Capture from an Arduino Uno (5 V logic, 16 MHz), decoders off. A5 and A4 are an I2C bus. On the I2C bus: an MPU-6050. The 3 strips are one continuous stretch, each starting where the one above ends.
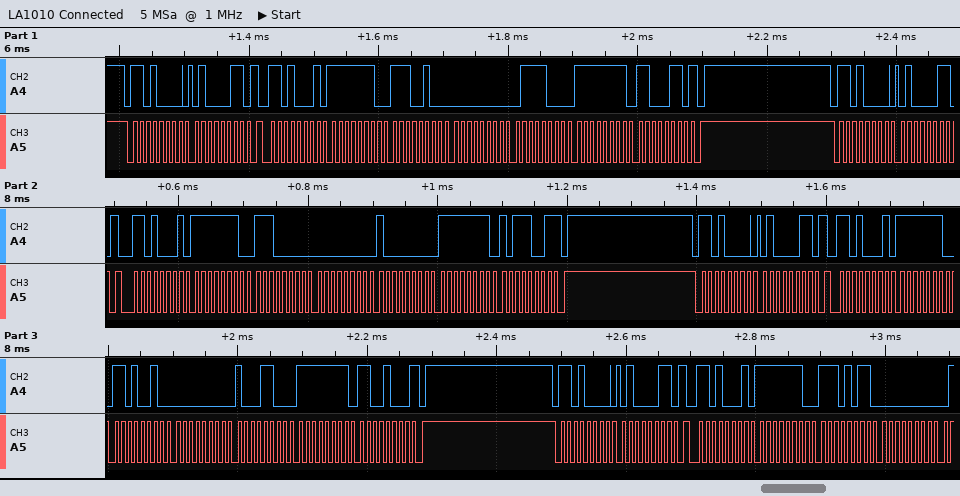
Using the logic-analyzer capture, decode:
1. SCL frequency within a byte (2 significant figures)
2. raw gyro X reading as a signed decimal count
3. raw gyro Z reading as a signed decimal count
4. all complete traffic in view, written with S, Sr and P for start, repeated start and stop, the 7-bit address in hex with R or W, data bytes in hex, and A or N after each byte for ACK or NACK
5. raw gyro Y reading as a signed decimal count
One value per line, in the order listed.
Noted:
100 kHz
-284
-58
S 68W A 43 A Sr 68R A FE A E4 A 00 A 78 A FF A C6 N P S 68W A 43 A Sr 68R A FE A E0 A 00 A 80 A FF A B9 N P S 68W A 43 A Sr 68R A FE A D2 A 00 A 8C A FF A C8 N P S 68W A 43 A Sr 68R A FE A EB A 00 A
120
